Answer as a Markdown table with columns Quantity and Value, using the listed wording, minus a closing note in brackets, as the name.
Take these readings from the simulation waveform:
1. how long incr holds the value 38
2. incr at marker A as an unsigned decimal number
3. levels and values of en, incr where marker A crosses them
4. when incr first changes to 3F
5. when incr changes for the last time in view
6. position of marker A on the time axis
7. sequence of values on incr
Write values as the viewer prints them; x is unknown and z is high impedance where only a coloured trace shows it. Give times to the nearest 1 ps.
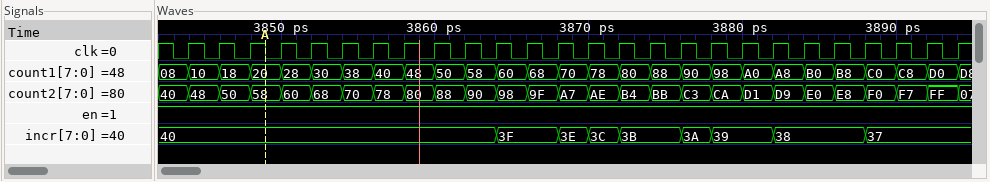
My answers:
| Quantity | Value |
|---|---|
| how long incr holds the value 38 | 6 ps |
| incr at marker A as an unsigned decimal number | 64 |
| levels and values of en, incr where marker A crosses them | en=1, incr=40 |
| when incr first changes to 3F | 3864 ps |
| when incr changes for the last time in view | 3888 ps |
| position of marker A on the time axis | 3849 ps |
| sequence of values on incr | 40, 3F, 3E, 3C, 3B, 3A, 39, 38, 37 |
